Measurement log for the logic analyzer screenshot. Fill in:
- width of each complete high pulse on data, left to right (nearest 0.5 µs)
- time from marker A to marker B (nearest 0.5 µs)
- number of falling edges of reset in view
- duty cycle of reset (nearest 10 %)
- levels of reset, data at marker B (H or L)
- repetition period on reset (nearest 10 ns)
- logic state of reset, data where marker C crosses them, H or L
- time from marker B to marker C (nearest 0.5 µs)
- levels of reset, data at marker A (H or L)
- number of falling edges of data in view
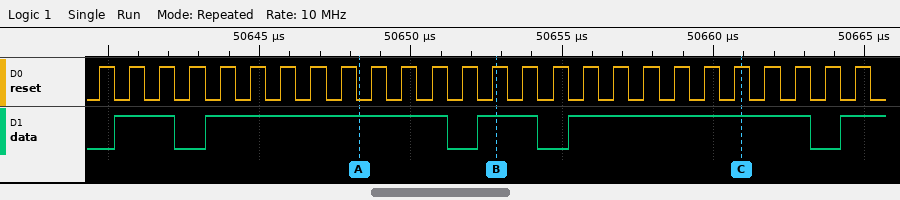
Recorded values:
2 µs, 8 µs, 2 µs, 8 µs
4.5 µs
26
50 %
reset=H, data=H
1000 ns
reset=H, data=H
8 µs
reset=L, data=H
4
